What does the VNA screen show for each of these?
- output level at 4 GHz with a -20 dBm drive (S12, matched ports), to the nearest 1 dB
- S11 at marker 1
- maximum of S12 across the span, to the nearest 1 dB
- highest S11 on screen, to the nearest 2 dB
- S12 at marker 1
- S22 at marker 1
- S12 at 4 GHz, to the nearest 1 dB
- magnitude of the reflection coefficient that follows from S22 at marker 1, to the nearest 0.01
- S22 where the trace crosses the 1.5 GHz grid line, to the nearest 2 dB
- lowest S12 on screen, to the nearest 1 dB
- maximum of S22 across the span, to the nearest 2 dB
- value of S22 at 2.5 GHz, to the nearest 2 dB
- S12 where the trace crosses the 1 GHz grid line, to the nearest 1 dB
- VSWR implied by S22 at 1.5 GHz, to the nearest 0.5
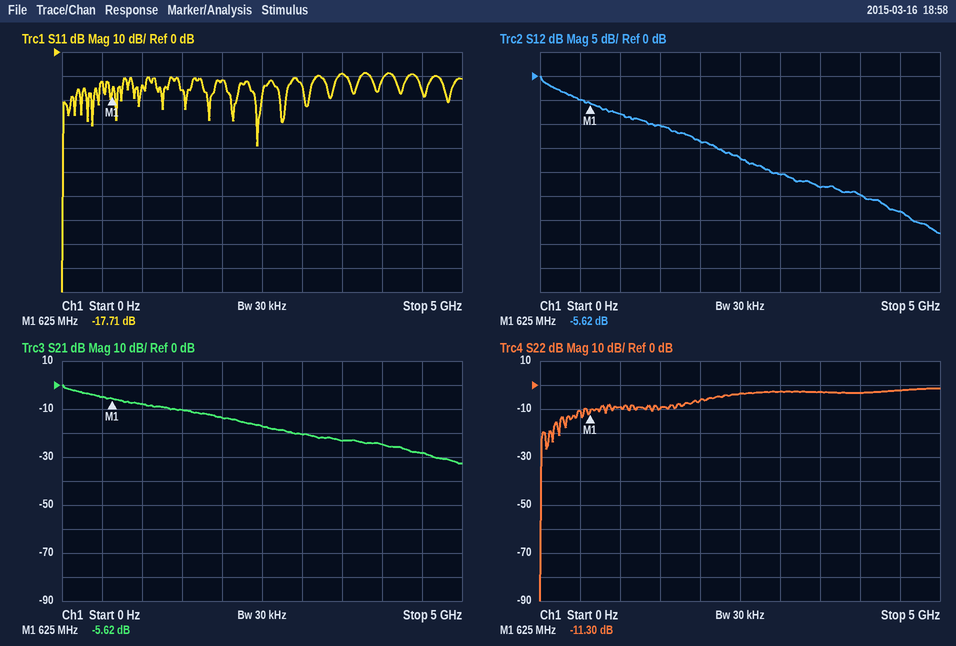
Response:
-45 dBm
-17.71 dB
0 dB
-8 dB
-5.62 dB
-11.30 dB
-25 dB
0.27
-10 dB
-33 dB
-2 dB
-4 dB
-8 dB
2.0
